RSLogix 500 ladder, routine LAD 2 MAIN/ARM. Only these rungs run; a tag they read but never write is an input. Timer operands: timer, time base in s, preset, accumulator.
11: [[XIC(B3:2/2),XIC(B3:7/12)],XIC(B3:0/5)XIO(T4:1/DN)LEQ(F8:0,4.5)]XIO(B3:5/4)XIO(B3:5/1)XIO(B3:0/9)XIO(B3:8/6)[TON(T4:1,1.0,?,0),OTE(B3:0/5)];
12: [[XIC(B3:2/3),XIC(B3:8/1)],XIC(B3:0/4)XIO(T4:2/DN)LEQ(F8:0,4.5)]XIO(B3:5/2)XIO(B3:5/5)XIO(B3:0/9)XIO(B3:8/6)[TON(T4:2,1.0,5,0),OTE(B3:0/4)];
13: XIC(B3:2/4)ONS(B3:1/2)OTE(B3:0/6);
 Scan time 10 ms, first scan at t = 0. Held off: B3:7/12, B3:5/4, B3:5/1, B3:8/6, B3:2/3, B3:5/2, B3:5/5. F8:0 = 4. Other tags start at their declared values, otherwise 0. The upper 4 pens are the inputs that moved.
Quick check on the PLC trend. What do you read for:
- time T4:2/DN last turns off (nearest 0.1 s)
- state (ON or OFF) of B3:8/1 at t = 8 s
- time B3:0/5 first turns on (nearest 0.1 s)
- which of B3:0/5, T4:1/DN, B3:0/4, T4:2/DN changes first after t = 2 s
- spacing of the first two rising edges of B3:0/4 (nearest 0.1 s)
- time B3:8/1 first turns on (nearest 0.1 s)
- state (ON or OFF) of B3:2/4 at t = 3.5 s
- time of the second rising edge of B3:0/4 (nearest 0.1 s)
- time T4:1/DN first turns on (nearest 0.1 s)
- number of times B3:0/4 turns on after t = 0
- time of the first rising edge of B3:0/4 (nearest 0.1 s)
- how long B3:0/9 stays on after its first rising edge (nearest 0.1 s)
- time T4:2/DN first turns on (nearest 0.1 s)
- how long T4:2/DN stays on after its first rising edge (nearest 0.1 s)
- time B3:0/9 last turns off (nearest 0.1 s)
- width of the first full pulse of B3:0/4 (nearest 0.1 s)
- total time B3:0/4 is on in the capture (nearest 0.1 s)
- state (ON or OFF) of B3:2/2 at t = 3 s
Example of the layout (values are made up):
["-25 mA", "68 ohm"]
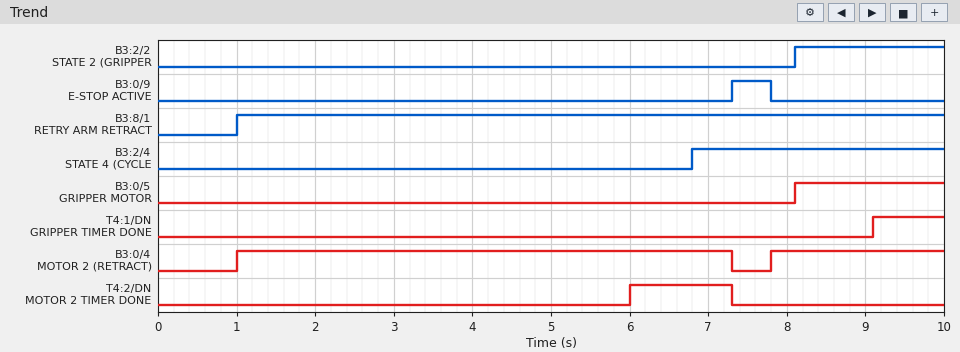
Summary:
["7.3 s", "ON", "8.1 s", "T4:2/DN", "6.8 s", "1.0 s", "OFF", "7.8 s", "9.1 s", "2", "1.0 s", "0.5 s", "6.0 s", "1.3 s", "7.8 s", "6.3 s", "8.5 s", "OFF"]
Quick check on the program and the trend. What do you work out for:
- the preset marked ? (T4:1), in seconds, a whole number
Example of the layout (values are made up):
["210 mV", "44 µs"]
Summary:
["1 s"]
